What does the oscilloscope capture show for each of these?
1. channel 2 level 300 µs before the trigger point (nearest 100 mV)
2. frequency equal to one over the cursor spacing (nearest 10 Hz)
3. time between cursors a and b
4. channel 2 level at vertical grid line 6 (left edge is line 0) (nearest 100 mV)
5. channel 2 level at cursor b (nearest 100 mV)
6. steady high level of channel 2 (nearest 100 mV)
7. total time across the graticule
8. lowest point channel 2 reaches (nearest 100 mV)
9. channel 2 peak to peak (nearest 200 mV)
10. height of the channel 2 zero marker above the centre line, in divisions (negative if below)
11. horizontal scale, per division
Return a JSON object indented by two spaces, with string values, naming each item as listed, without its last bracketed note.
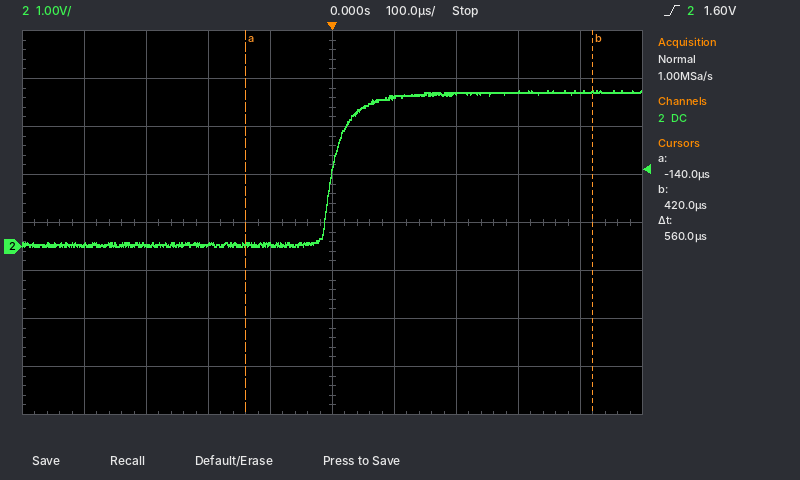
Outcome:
{
  "channel 2 level 300 µs before the trigger point": "0.0 V",
  "frequency equal to one over the cursor spacing": "1.79 kHz",
  "time between cursors a and b": "560 µs",
  "channel 2 level at vertical grid line 6 (left edge is line 0)": "3.1 V",
  "channel 2 level at cursor b": "3.2 V",
  "steady high level of channel 2": "3.2 V",
  "total time across the graticule": "1 ms",
  "lowest point channel 2 reaches": "0.0 V",
  "channel 2 peak to peak": "3.2 V",
  "height of the channel 2 zero marker above the centre line, in divisions": "-0.5 div",
  "horizontal scale, per division": "100 µs"
}
